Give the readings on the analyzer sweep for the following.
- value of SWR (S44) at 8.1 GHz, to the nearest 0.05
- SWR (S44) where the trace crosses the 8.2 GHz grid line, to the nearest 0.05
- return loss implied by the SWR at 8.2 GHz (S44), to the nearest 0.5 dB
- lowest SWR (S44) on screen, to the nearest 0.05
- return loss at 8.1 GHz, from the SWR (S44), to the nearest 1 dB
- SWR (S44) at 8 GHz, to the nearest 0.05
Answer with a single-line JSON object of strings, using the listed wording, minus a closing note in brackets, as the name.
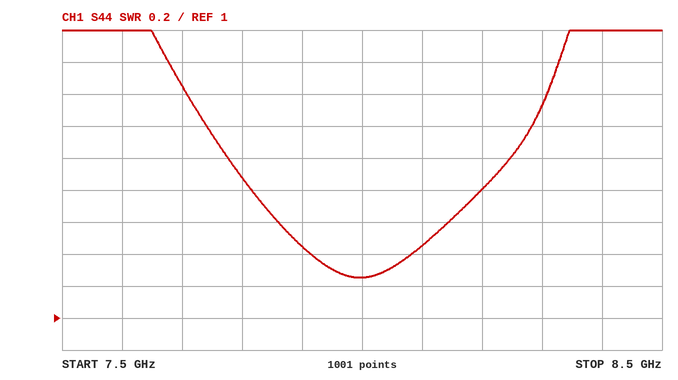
{"value of SWR (S44) at 8.1 GHz, to the nearest 0.05": "1.45", "SWR (S44) where the trace crosses the 8.2 GHz grid line, to the nearest 0.05": "1.80", "return loss implied by the SWR at 8.2 GHz (S44), to the nearest 0.5 dB": "11.0 dB", "lowest SWR (S44) on screen, to the nearest 0.05": "1.25", "return loss at 8.1 GHz, from the SWR (S44), to the nearest 1 dB": "15 dB", "SWR (S44) at 8 GHz, to the nearest 0.05": "1.25"}
